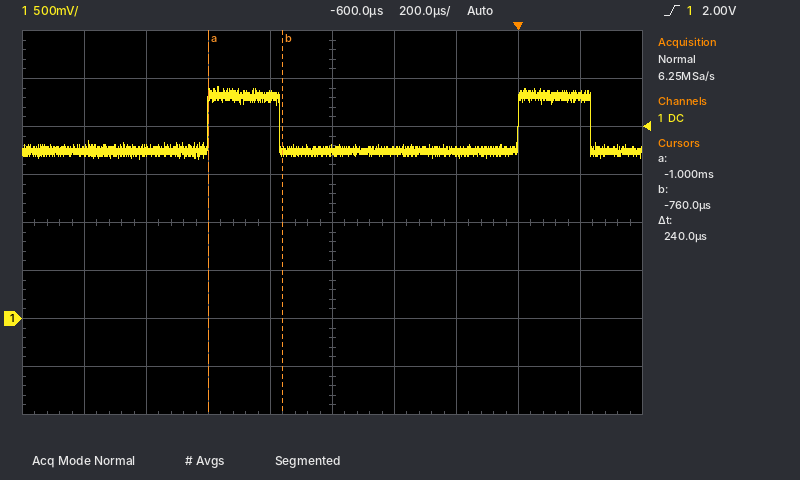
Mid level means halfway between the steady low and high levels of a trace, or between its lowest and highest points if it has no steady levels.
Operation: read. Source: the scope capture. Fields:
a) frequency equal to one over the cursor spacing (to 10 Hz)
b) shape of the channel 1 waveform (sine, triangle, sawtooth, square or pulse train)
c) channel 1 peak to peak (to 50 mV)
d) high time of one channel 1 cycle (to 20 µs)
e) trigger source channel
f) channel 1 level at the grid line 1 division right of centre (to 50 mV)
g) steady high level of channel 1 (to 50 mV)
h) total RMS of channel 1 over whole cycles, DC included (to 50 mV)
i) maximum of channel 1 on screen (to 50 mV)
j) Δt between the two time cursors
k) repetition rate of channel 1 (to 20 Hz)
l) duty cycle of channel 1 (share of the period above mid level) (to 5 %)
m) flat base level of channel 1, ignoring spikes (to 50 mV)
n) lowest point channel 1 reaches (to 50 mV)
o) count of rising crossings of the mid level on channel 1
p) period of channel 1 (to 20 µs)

4.17 kHz
pulse train
750 mV
240 µs
channel 1
1.75 V
2.30 V
1.90 V
2.40 V
240 µs
1.00 kHz
25 %
1.75 V
1.65 V
2
1.00 ms
